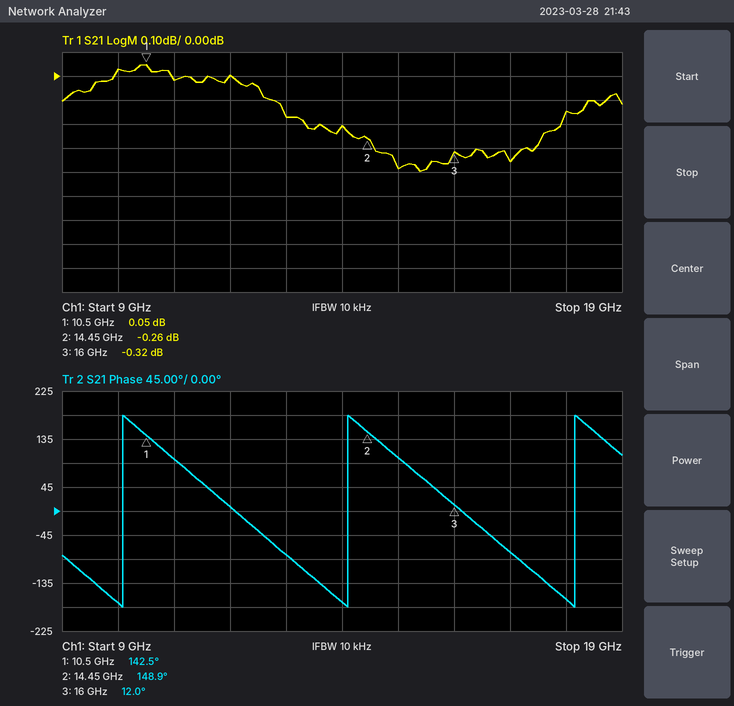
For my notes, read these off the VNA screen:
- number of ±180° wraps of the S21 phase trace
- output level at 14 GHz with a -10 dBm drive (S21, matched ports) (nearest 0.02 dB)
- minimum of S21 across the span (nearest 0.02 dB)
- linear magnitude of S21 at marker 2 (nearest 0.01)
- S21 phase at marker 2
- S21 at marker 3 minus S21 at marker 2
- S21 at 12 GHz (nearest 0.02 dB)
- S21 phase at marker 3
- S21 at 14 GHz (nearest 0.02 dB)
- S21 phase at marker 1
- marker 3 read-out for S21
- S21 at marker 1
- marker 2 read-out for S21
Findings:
3
-10.20 dBm
-0.40 dB
0.97
148.9°
-0.06 dB
0.00 dB
12.0°
-0.20 dB
142.5°
-0.32 dB
0.05 dB
-0.26 dB
